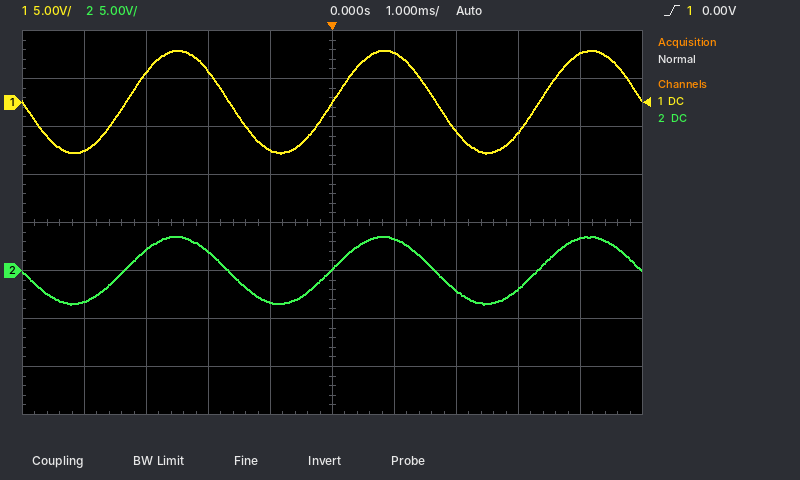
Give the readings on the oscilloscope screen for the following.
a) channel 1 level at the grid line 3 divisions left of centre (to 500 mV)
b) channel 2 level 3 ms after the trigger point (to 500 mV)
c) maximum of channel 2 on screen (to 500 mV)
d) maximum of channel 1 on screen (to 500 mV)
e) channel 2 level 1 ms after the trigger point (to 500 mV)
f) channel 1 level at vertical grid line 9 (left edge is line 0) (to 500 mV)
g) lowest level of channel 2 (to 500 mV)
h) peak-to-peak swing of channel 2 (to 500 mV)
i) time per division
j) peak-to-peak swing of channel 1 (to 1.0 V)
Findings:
3.0 V
-2.0 V
3.5 V
5.5 V
3.5 V
5.0 V
-3.5 V
7.0 V
1 ms
11.0 V
